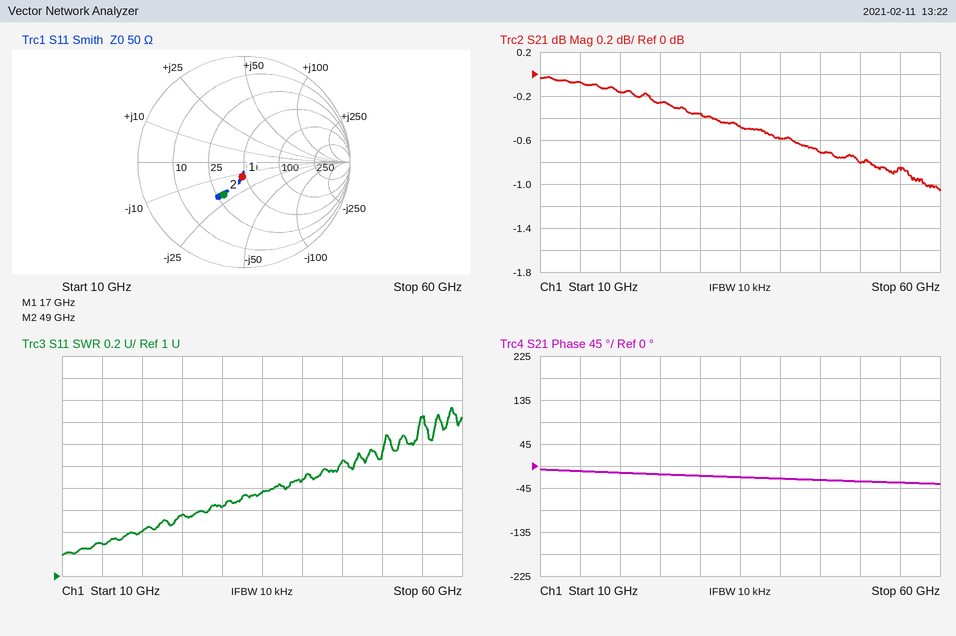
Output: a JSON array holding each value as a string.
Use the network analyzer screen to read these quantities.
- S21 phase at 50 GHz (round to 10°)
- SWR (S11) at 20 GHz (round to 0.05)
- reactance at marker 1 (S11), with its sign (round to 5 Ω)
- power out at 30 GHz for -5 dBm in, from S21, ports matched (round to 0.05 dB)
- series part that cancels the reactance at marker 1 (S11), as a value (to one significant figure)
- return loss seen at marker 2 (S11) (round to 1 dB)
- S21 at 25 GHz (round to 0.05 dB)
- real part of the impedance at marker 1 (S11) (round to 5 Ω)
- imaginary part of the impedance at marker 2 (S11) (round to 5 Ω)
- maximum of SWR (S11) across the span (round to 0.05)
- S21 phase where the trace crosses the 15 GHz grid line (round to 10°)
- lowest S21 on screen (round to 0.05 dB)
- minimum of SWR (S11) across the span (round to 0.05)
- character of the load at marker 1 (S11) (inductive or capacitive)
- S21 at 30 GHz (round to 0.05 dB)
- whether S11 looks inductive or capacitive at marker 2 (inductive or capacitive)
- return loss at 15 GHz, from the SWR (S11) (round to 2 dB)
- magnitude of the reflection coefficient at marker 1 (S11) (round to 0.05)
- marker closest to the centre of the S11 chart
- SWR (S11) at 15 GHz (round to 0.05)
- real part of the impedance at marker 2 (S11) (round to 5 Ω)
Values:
["-30°", "1.40", "-15 Ω", "-5.35 dBm", "100 pH", "9 dB", "-0.25 dB", "45 Ω", "-20 Ω", "2.55", "-10°", "-1.05 dB", "1.20", "capacitive", "-0.35 dB", "capacitive", "18 dB", "0.15", "marker 1", "1.30", "30 Ω"]
